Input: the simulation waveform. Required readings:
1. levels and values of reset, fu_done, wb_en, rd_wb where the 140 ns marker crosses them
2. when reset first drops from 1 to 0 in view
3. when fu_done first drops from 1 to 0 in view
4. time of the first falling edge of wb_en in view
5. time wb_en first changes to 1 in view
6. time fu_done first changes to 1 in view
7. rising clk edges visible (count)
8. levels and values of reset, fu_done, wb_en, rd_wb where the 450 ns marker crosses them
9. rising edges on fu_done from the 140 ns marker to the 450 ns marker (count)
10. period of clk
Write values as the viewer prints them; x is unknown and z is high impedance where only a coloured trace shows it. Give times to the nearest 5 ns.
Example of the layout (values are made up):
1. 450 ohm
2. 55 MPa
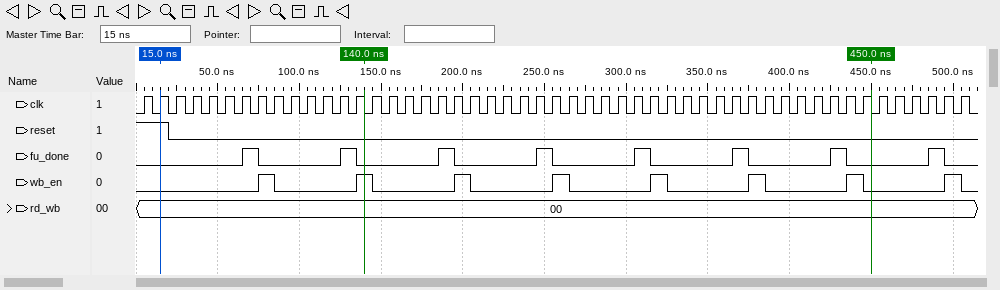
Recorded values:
1. reset=0, fu_done=0, wb_en=1, rd_wb=00
2. 20 ns
3. 75 ns
4. 85 ns
5. 75 ns
6. 65 ns
7. 51
8. reset=0, fu_done=0, wb_en=0, rd_wb=00
9. 5
10. 10 ns
